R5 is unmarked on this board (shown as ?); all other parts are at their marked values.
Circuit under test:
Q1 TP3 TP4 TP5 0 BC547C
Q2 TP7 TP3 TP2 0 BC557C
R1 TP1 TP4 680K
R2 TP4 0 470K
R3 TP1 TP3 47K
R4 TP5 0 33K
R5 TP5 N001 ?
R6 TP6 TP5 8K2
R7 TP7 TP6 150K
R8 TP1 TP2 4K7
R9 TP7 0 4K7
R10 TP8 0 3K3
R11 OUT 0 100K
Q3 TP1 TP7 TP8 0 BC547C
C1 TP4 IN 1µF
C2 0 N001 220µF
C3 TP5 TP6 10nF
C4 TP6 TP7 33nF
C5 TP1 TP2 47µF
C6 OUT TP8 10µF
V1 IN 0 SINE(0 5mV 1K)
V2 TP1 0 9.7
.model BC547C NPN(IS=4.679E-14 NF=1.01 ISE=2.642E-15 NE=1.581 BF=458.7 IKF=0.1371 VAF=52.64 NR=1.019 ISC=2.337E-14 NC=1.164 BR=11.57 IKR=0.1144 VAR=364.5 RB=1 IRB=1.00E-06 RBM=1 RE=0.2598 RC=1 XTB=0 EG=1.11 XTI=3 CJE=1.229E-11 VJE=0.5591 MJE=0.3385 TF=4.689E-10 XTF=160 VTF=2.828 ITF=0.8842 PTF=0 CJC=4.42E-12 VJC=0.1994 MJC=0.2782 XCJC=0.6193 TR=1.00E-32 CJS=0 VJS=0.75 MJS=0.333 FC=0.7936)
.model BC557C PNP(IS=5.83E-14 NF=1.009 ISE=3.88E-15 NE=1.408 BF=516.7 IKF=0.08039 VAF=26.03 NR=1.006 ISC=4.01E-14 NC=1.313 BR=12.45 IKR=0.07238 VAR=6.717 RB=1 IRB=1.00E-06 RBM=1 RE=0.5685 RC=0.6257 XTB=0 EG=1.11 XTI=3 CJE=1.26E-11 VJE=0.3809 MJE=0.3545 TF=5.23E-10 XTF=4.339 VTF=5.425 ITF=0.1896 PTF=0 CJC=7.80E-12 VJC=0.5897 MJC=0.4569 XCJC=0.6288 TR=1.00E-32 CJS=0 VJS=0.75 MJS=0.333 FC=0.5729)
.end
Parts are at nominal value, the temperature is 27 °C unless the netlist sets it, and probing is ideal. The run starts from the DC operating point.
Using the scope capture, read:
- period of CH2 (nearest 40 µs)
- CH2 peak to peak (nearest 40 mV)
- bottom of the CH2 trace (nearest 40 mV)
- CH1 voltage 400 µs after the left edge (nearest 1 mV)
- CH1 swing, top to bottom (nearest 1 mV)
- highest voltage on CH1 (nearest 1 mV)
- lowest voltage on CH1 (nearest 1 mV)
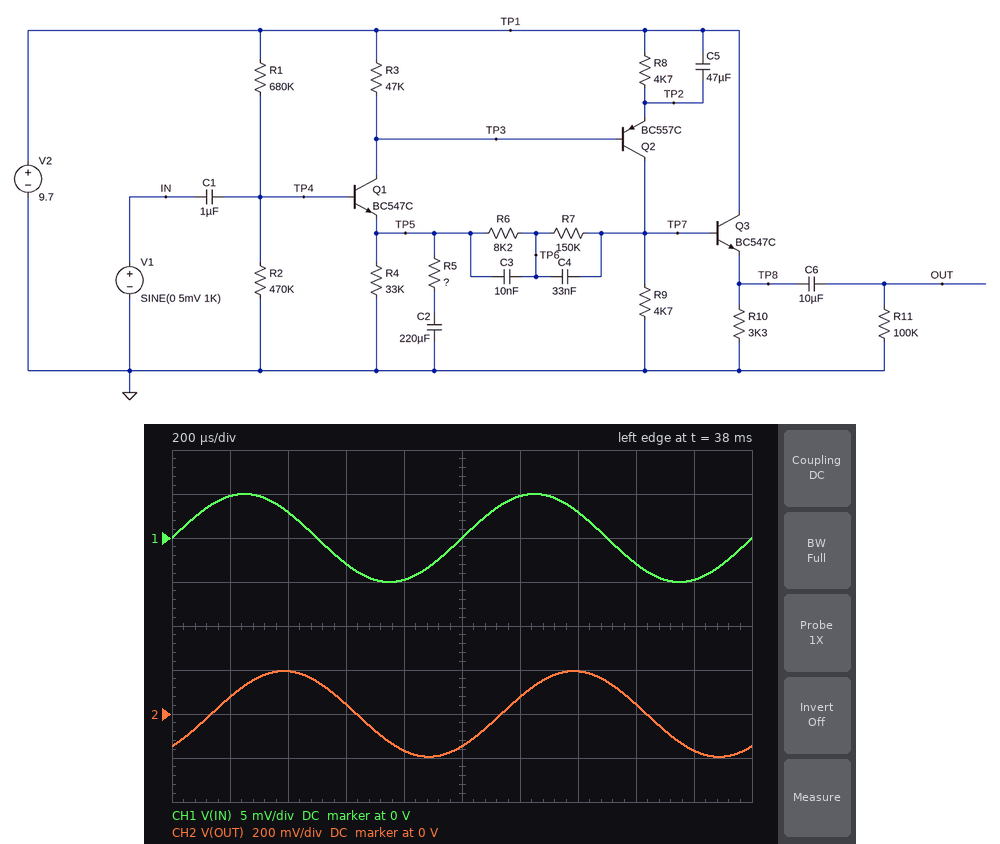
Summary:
1.00 ms
400 mV
-200 mV
3 mV
10 mV
5 mV
-5 mV
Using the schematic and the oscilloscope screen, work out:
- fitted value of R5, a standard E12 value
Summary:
270 Ω
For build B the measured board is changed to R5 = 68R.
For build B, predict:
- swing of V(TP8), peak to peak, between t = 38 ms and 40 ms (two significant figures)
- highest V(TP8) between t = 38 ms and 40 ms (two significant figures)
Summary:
1.5 V
4.0 V
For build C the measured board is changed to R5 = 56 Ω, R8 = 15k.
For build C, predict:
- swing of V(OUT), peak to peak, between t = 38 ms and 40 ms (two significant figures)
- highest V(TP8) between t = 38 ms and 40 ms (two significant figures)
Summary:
1.7 V
1.8 V
